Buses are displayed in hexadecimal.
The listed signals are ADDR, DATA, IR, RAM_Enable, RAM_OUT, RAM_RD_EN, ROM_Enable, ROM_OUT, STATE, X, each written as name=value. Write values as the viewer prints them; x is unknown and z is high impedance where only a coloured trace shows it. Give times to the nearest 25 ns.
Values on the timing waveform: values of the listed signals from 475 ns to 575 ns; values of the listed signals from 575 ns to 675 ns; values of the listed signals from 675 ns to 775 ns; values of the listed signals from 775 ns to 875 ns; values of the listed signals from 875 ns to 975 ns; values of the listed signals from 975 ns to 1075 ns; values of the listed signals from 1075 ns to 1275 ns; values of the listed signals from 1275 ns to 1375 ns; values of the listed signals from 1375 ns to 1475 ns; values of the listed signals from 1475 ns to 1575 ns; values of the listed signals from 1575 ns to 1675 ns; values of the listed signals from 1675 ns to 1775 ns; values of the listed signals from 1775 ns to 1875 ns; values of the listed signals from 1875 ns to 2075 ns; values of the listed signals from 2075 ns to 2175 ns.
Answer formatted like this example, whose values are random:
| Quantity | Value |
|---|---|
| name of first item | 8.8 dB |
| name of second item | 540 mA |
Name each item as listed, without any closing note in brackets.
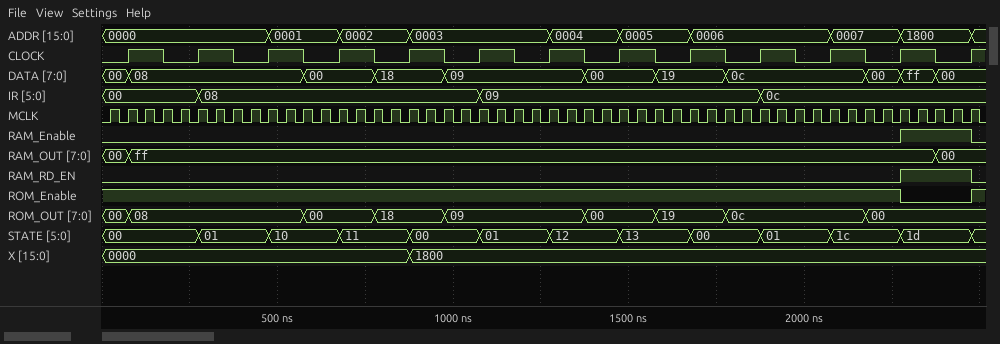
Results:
| Quantity | Value |
|---|---|
| values of the listed signals from 475 ns to 575 ns | ADDR=0001, DATA=08, IR=08, RAM_Enable=0, RAM_OUT=ff, RAM_RD_EN=0, ROM_Enable=1, ROM_OUT=08, STATE=10, X=0000 |
| values of the listed signals from 575 ns to 675 ns | ADDR=0001, DATA=00, IR=08, RAM_Enable=0, RAM_OUT=ff, RAM_RD_EN=0, ROM_Enable=1, ROM_OUT=00, STATE=10, X=0000 |
| values of the listed signals from 675 ns to 775 ns | ADDR=0002, DATA=00, IR=08, RAM_Enable=0, RAM_OUT=ff, RAM_RD_EN=0, ROM_Enable=1, ROM_OUT=00, STATE=11, X=0000 |
| values of the listed signals from 775 ns to 875 ns | ADDR=0002, DATA=18, IR=08, RAM_Enable=0, RAM_OUT=ff, RAM_RD_EN=0, ROM_Enable=1, ROM_OUT=18, STATE=11, X=0000 |
| values of the listed signals from 875 ns to 975 ns | ADDR=0003, DATA=18, IR=08, RAM_Enable=0, RAM_OUT=ff, RAM_RD_EN=0, ROM_Enable=1, ROM_OUT=18, STATE=00, X=1800 |
| values of the listed signals from 975 ns to 1075 ns | ADDR=0003, DATA=09, IR=08, RAM_Enable=0, RAM_OUT=ff, RAM_RD_EN=0, ROM_Enable=1, ROM_OUT=09, STATE=00, X=1800 |
| values of the listed signals from 1075 ns to 1275 ns | ADDR=0003, DATA=09, IR=09, RAM_Enable=0, RAM_OUT=ff, RAM_RD_EN=0, ROM_Enable=1, ROM_OUT=09, STATE=01, X=1800 |
| values of the listed signals from 1275 ns to 1375 ns | ADDR=0004, DATA=09, IR=09, RAM_Enable=0, RAM_OUT=ff, RAM_RD_EN=0, ROM_Enable=1, ROM_OUT=09, STATE=12, X=1800 |
| values of the listed signals from 1375 ns to 1475 ns | ADDR=0004, DATA=00, IR=09, RAM_Enable=0, RAM_OUT=ff, RAM_RD_EN=0, ROM_Enable=1, ROM_OUT=00, STATE=12, X=1800 |
| values of the listed signals from 1475 ns to 1575 ns | ADDR=0005, DATA=00, IR=09, RAM_Enable=0, RAM_OUT=ff, RAM_RD_EN=0, ROM_Enable=1, ROM_OUT=00, STATE=13, X=1800 |
| values of the listed signals from 1575 ns to 1675 ns | ADDR=0005, DATA=19, IR=09, RAM_Enable=0, RAM_OUT=ff, RAM_RD_EN=0, ROM_Enable=1, ROM_OUT=19, STATE=13, X=1800 |
| values of the listed signals from 1675 ns to 1775 ns | ADDR=0006, DATA=19, IR=09, RAM_Enable=0, RAM_OUT=ff, RAM_RD_EN=0, ROM_Enable=1, ROM_OUT=19, STATE=00, X=1800 |
| values of the listed signals from 1775 ns to 1875 ns | ADDR=0006, DATA=0c, IR=09, RAM_Enable=0, RAM_OUT=ff, RAM_RD_EN=0, ROM_Enable=1, ROM_OUT=0c, STATE=00, X=1800 |
| values of the listed signals from 1875 ns to 2075 ns | ADDR=0006, DATA=0c, IR=0c, RAM_Enable=0, RAM_OUT=ff, RAM_RD_EN=0, ROM_Enable=1, ROM_OUT=0c, STATE=01, X=1800 |
| values of the listed signals from 2075 ns to 2175 ns | ADDR=0007, DATA=0c, IR=0c, RAM_Enable=0, RAM_OUT=ff, RAM_RD_EN=0, ROM_Enable=1, ROM_OUT=0c, STATE=1c, X=1800 |
